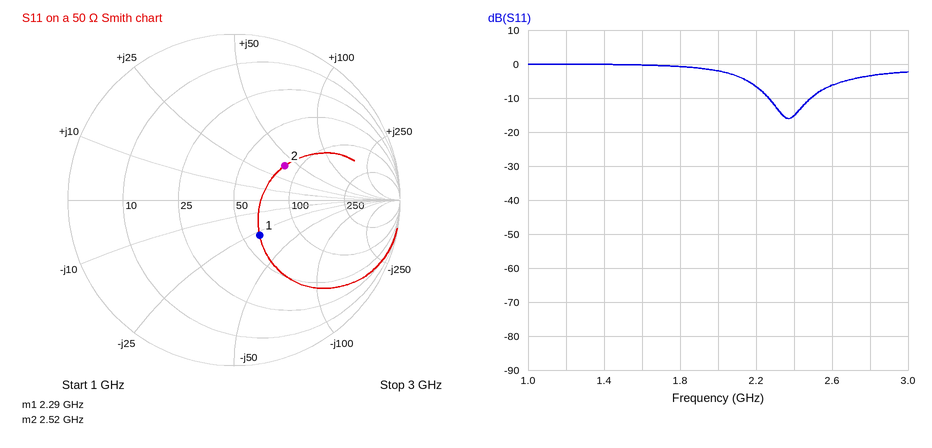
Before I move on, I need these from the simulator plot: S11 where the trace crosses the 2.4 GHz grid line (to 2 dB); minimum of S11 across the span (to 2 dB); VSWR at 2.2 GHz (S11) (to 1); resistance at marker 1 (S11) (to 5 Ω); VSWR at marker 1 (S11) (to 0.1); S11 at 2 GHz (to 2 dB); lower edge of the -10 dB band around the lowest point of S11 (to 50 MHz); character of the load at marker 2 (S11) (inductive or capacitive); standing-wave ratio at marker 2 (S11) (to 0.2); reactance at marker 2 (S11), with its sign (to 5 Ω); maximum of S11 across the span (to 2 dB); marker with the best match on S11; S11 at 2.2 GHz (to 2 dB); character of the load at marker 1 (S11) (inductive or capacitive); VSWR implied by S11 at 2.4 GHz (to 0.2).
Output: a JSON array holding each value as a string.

["-16 dB", "-16 dB", "3", "60 Ω", "1.7", "-2 dB", "2.25 GHz", "inductive", "2.2", "+40 Ω", "0 dB", "marker 1", "-6 dB", "capacitive", "1.4"]
